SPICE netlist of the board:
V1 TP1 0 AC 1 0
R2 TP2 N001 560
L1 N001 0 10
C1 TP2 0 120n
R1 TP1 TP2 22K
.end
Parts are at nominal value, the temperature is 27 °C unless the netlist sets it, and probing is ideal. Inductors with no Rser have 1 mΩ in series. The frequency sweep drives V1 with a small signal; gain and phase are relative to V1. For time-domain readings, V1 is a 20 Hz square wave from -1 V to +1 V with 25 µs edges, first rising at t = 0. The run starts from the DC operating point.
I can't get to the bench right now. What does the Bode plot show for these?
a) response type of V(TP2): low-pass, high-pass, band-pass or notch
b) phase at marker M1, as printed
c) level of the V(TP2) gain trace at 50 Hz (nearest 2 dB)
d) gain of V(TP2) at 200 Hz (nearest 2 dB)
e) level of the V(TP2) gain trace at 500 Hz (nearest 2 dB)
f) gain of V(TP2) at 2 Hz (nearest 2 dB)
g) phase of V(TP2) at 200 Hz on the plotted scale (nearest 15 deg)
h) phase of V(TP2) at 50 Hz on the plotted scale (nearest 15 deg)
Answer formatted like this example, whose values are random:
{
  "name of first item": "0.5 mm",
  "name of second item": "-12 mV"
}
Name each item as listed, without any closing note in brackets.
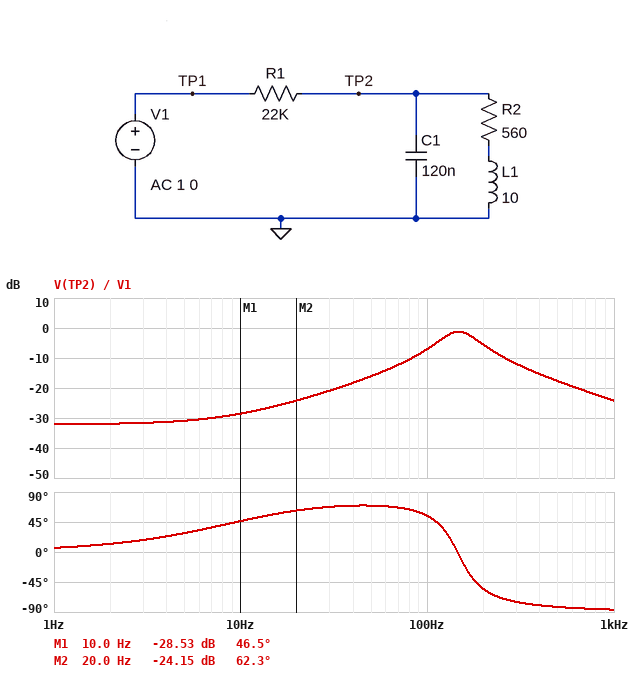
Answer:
{
  "response type of V(TP2): low-pass, high-pass, band-pass or notch": "band-pass",
  "phase at marker M1, as printed": "46.5 deg",
  "level of the V(TP2) gain trace at 50 Hz": "-16 dB",
  "gain of V(TP2) at 200 Hz": "-6 dB",
  "level of the V(TP2) gain trace at 500 Hz": "-18 dB",
  "gain of V(TP2) at 2 Hz": "-32 dB",
  "phase of V(TP2) at 200 Hz on the plotted scale": "-60 deg",
  "phase of V(TP2) at 50 Hz on the plotted scale": "75 deg"
}
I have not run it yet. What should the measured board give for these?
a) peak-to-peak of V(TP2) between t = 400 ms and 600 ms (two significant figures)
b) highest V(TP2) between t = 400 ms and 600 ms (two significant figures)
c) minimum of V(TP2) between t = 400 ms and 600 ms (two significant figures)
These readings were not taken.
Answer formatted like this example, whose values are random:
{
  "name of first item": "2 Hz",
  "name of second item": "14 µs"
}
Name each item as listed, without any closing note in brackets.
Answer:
{
  "peak-to-peak of V(TP2) between t = 400 ms and 600 ms": "1.2 V",
  "highest V(TP2) between t = 400 ms and 600 ms": "610 mV",
  "minimum of V(TP2) between t = 400 ms and 600 ms": "-610 mV"
}
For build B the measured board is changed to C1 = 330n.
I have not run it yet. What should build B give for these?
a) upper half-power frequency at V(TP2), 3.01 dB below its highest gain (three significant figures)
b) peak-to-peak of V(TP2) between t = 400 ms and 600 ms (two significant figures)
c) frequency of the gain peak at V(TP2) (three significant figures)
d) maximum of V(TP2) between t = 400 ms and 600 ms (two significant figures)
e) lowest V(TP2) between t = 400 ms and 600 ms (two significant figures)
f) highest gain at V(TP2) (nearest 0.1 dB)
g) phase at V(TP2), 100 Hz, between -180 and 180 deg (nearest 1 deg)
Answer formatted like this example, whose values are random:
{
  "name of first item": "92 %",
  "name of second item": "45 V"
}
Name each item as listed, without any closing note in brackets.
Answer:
{
  "upper half-power frequency at V(TP2), 3.01 dB below its highest gain": "105 Hz",
  "peak-to-peak of V(TP2) between t = 400 ms and 600 ms": "760 mV",
  "frequency of the gain peak at V(TP2)": "88.7 Hz",
  "maximum of V(TP2) between t = 400 ms and 600 ms": "380 mV",
  "lowest V(TP2) between t = 400 ms and 600 ms": "-380 mV",
  "highest gain at V(TP2)": "-2.9 dB",
  "phase at V(TP2), 100 Hz, between -180 and 180 deg": "-40 deg"
}
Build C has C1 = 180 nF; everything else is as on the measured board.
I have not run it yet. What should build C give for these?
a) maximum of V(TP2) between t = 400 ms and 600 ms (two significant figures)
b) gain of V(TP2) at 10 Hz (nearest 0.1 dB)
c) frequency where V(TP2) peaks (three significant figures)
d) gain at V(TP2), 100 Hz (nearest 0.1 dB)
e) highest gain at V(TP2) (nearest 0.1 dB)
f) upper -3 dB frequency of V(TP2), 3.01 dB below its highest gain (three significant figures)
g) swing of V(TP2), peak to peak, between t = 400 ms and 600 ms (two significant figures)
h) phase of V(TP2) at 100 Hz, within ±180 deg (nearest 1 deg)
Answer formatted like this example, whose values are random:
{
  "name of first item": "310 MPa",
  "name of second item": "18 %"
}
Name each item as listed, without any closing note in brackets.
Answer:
{
  "maximum of V(TP2) between t = 400 ms and 600 ms": "510 mV",
  "gain of V(TP2) at 10 Hz": "-28.5 dB",
  "frequency where V(TP2) peaks": "120 Hz",
  "gain at V(TP2), 100 Hz": "-4.3 dB",
  "highest gain at V(TP2)": "-1.7 dB",
  "upper -3 dB frequency of V(TP2), 3.01 dB below its highest gain": "147 Hz",
  "swing of V(TP2), peak to peak, between t = 400 ms and 600 ms": "1.0 V",
  "phase of V(TP2) at 100 Hz, within ±180 deg": "37 deg"
}
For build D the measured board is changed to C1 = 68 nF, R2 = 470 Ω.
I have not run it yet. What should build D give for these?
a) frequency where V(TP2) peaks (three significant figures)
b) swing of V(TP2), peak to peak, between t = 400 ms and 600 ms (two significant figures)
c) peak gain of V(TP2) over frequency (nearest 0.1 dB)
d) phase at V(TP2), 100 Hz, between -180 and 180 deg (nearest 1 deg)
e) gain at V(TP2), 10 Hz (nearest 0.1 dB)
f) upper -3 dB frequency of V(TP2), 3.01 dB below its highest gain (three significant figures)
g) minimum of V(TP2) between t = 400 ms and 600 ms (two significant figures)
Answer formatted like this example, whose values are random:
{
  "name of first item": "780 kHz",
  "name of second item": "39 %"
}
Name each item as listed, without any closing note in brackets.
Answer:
{
  "frequency where V(TP2) peaks": "195 Hz",
  "swing of V(TP2), peak to peak, between t = 400 ms and 600 ms": "1.5 V",
  "peak gain of V(TP2) over frequency": "-0.6 dB",
  "phase at V(TP2), 100 Hz, between -180 and 180 deg": "64 deg",
  "gain at V(TP2), 10 Hz": "-29.1 dB",
  "upper -3 dB frequency of V(TP2), 3.01 dB below its highest gain": "260 Hz",
  "minimum of V(TP2) between t = 400 ms and 600 ms": "-750 mV"
}
